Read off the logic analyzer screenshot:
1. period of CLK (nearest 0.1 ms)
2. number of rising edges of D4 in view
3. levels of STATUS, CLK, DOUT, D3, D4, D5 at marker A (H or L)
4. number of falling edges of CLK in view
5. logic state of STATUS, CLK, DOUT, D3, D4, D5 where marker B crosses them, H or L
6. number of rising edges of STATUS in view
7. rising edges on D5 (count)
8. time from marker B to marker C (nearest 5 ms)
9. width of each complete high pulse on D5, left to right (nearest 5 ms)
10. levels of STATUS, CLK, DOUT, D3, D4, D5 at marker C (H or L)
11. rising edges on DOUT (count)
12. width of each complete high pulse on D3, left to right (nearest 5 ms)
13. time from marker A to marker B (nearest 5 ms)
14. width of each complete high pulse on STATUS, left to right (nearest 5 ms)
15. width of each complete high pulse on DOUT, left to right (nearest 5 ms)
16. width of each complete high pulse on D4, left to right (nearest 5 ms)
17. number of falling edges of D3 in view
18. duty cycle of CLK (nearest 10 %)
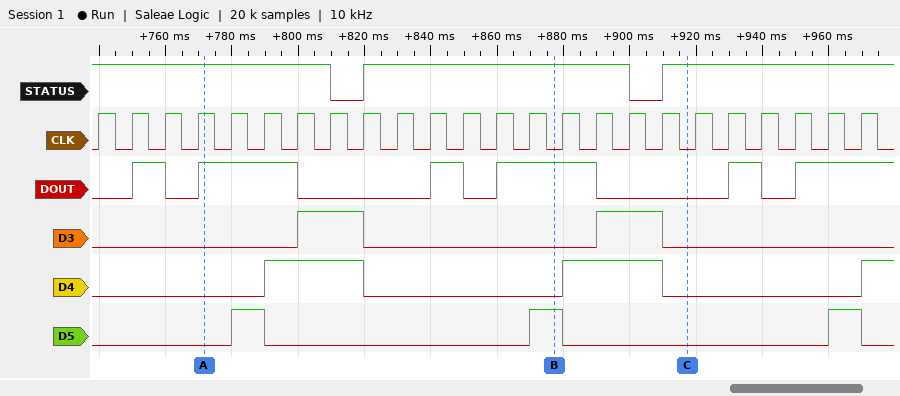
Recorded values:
10 ms
3
STATUS=H, CLK=H, DOUT=H, D3=L, D4=L, D5=L
24
STATUS=H, CLK=L, DOUT=H, D3=L, D4=L, D5=H
2
3
40 ms
10 ms, 10 ms, 10 ms
STATUS=H, CLK=L, DOUT=L, D3=L, D4=L, D5=L
6
20 ms, 20 ms
105 ms
80 ms
10 ms, 30 ms, 10 ms, 30 ms, 10 ms
30 ms, 30 ms
2
50 %
